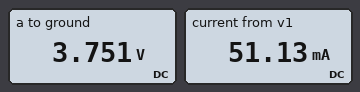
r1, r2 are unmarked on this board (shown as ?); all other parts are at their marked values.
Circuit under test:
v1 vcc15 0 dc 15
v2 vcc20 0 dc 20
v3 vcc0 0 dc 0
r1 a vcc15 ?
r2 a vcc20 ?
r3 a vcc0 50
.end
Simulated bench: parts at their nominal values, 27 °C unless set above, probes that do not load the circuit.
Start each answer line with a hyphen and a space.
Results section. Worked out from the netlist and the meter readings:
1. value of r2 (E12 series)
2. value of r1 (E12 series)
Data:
- 680 Ω
- 220 Ω
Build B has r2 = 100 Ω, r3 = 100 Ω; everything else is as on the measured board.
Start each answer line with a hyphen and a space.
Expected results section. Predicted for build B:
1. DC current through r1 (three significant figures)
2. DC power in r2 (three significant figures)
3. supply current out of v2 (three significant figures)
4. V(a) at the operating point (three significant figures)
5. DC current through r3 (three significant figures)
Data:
- 18.5 mA
- 823 mW
- 90.7 mA
- 10.9 V
- 109 mA
